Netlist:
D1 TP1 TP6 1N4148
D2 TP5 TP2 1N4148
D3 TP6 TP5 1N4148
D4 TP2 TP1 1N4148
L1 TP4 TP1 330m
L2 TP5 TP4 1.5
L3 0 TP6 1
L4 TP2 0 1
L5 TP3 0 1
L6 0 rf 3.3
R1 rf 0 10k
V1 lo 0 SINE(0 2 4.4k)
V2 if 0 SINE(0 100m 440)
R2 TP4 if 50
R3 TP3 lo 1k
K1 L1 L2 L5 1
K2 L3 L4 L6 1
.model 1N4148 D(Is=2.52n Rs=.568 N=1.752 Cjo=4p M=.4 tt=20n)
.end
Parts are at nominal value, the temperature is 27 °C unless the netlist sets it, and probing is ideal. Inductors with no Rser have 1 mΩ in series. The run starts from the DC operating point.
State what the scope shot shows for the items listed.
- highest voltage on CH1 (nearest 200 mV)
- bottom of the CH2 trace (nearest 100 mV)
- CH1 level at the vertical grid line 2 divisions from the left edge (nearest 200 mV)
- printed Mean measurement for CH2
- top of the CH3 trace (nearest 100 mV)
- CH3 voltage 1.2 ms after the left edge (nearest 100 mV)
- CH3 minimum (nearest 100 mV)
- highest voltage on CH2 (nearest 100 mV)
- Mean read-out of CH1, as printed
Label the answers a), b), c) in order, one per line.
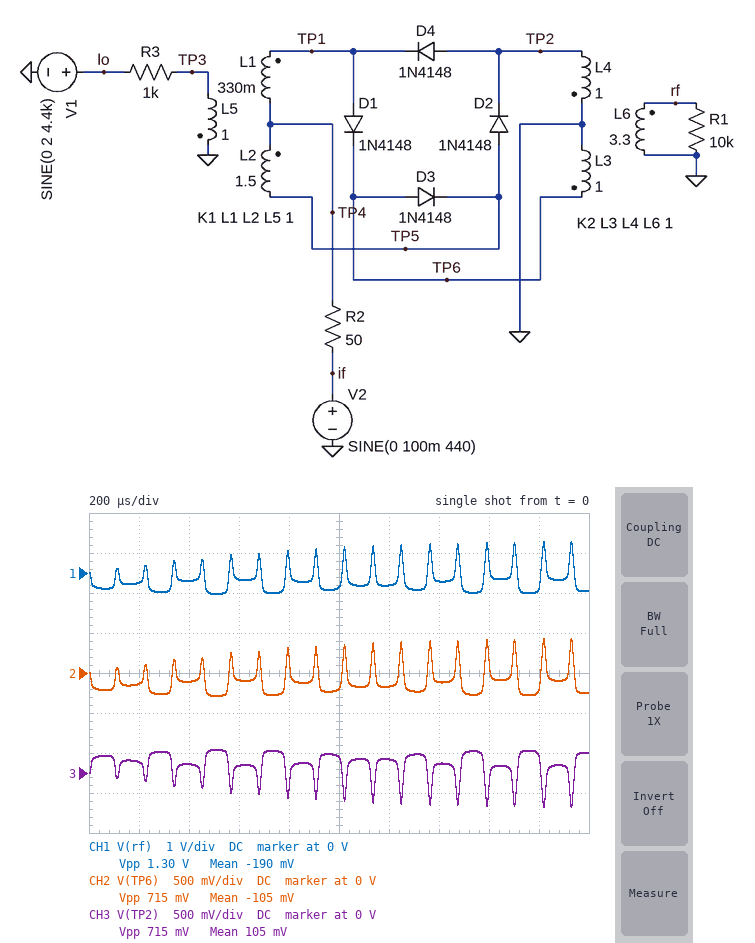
a) 800 mV
b) -300 mV
c) -200 mV
d) -105 mV
e) 300 mV
f) 200 mV
g) -400 mV
h) 400 mV
i) -190 mV
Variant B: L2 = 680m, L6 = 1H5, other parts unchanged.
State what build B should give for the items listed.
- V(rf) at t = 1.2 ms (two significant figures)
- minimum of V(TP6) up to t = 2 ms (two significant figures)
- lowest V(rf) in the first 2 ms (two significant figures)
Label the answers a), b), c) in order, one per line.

a) -97 mV
b) -200 mV
c) -240 mV
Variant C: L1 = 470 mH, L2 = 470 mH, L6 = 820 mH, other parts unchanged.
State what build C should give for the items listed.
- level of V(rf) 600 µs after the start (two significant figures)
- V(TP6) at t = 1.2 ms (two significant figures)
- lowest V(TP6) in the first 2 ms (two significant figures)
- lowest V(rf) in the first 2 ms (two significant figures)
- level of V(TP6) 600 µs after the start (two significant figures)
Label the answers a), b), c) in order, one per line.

a) 90 mV
b) 17 mV
c) -99 mV
d) -90 mV
e) 99 mV
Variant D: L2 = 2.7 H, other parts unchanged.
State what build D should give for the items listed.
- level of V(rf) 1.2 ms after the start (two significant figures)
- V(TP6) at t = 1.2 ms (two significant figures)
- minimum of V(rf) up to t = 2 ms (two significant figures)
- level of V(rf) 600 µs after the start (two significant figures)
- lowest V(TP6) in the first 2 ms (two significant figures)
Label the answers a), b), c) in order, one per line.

a) -410 mV
b) -230 mV
c) -640 mV
d) -270 mV
e) -350 mV
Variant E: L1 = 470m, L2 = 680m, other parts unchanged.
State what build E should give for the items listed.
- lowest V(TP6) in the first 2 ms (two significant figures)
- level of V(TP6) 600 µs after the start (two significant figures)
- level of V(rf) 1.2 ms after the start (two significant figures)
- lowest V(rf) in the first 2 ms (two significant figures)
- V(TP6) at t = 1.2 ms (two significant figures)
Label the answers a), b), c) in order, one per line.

a) -150 mV
b) 49 mV
c) -58 mV
d) -270 mV
e) -32 mV
